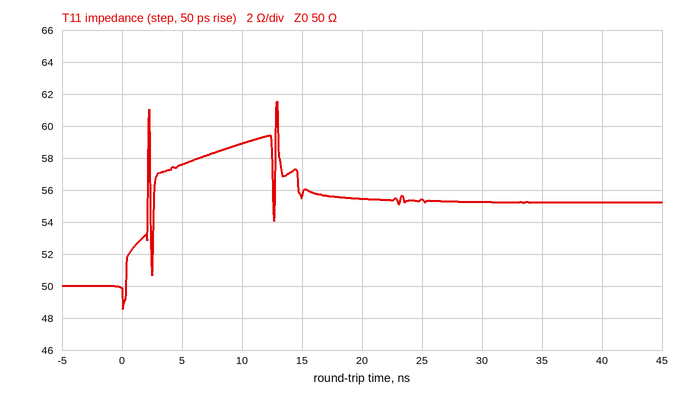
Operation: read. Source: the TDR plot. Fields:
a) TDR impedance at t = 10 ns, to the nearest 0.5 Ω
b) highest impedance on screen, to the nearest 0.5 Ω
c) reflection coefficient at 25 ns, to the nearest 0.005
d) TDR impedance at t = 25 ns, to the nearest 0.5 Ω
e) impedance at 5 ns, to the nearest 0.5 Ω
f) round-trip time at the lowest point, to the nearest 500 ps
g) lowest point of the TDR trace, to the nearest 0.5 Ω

59.0 Ω
61.5 Ω
+0.050
55.5 Ω
57.5 Ω
0.0 ns
48.5 Ω
